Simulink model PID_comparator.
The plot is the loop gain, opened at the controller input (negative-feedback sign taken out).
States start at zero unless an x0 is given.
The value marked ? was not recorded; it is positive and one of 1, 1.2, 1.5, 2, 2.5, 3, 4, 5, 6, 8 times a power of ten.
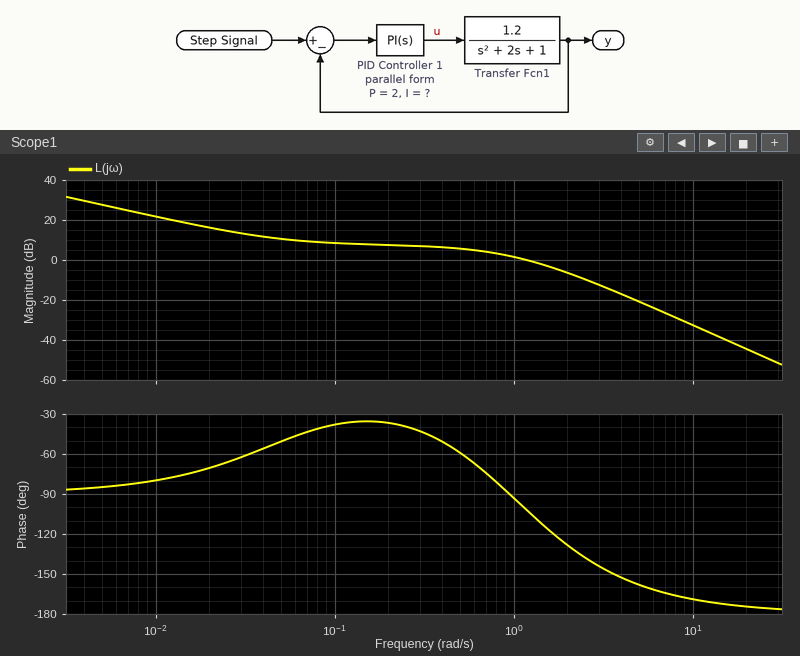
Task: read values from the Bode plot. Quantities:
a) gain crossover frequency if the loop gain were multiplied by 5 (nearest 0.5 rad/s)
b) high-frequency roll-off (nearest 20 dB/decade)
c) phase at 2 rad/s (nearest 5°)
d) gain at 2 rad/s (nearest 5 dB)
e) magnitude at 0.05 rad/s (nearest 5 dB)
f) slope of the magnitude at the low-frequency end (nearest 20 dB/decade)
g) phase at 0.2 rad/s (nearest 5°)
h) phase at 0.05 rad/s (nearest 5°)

3.5 rad/s
-40 dB/decade
-130°
-5 dB
10 dB
-20 dB/decade
-35°
-50°
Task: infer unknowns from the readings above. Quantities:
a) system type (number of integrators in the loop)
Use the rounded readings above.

1
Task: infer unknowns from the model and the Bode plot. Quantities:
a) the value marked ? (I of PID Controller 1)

0.1
